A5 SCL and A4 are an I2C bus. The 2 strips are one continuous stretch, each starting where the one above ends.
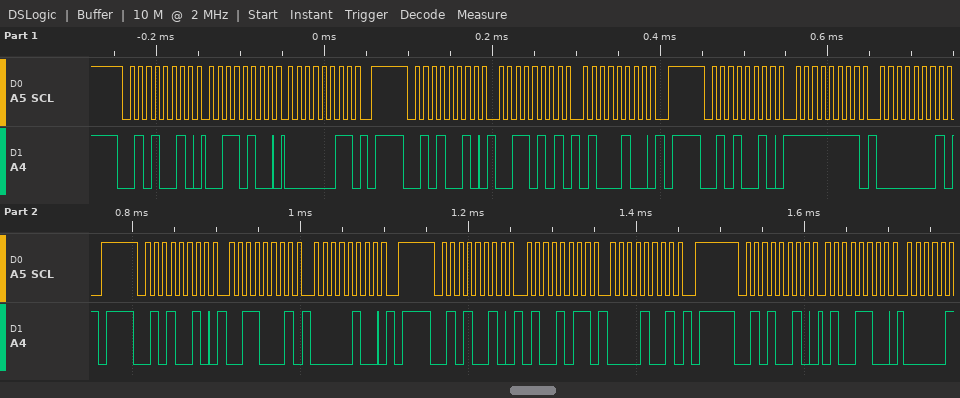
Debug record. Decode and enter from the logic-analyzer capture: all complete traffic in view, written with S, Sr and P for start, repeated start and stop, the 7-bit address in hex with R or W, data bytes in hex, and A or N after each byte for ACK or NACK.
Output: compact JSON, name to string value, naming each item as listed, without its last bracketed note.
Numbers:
{"all complete traffic in view, written with S, Sr and P for start, repeated start and stop, the 7-bit address in hex with R or W, data bytes in hex, and A or N after each byte for ACK or NACK": "S 29W A 34 A 03 A P S 29W A 35 A 44 A P S 29W A FF A 01 A P S 29W A 31 A 04 A P S 29W A 4B A 09 A P S 29W A 4C A"}
